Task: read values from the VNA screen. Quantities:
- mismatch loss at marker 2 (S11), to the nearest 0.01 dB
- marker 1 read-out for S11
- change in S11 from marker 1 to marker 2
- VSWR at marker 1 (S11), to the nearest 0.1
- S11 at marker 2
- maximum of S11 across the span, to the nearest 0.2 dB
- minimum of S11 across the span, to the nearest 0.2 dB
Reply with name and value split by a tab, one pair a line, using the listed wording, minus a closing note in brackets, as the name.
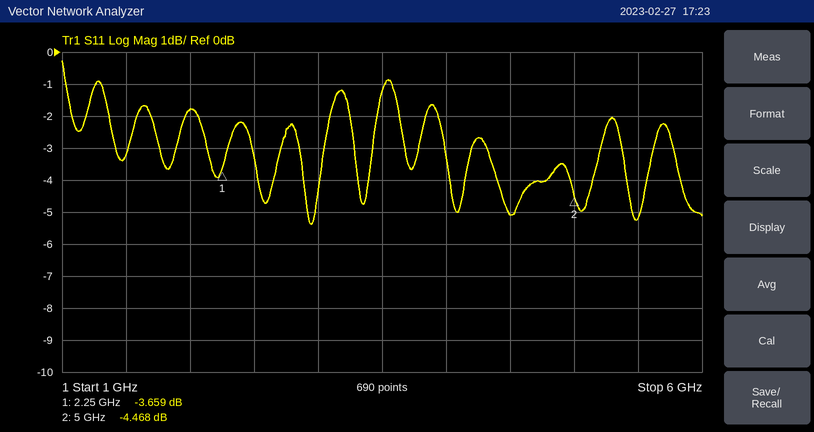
mismatch loss at marker 2 (S11), to the nearest 0.01 dB	1.92 dB
marker 1 read-out for S11	-3.659 dB
change in S11 from marker 1 to marker 2	-0.809 dB
VSWR at marker 1 (S11), to the nearest 0.1	4.8
S11 at marker 2	-4.468 dB
maximum of S11 across the span, to the nearest 0.2 dB	-0.2 dB
minimum of S11 across the span, to the nearest 0.2 dB	-5.4 dB
